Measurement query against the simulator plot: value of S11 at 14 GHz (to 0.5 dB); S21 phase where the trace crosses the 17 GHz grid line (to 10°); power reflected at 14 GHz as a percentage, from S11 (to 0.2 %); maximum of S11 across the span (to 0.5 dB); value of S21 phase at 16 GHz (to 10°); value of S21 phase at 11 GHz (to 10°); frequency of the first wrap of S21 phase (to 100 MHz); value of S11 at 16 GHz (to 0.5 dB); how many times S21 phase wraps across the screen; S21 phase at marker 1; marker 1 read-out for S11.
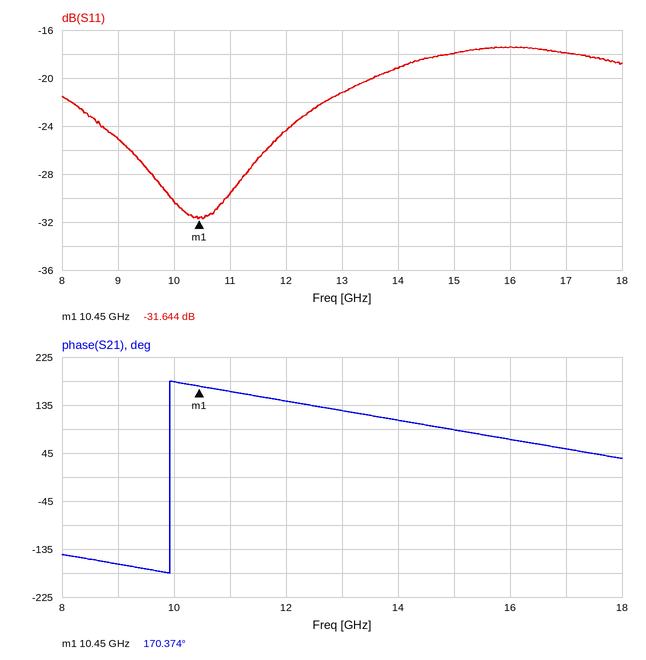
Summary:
-19.0 dB
50°
1.2 %
-17.5 dB
70°
160°
9.9 GHz
-17.5 dB
1
170.374°
-31.644 dB
